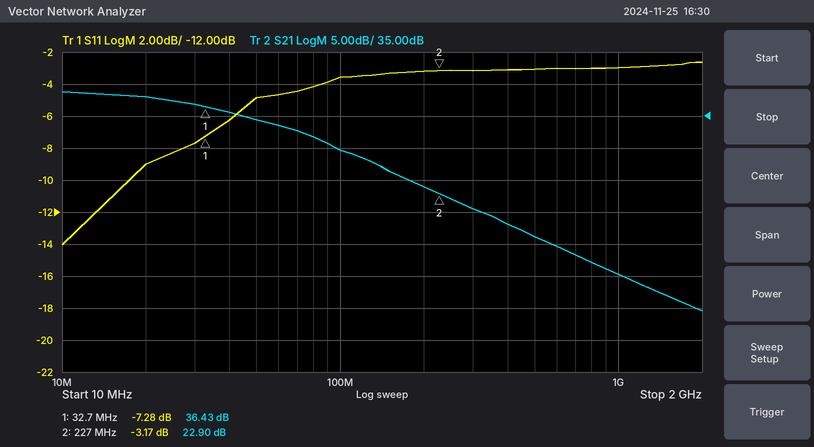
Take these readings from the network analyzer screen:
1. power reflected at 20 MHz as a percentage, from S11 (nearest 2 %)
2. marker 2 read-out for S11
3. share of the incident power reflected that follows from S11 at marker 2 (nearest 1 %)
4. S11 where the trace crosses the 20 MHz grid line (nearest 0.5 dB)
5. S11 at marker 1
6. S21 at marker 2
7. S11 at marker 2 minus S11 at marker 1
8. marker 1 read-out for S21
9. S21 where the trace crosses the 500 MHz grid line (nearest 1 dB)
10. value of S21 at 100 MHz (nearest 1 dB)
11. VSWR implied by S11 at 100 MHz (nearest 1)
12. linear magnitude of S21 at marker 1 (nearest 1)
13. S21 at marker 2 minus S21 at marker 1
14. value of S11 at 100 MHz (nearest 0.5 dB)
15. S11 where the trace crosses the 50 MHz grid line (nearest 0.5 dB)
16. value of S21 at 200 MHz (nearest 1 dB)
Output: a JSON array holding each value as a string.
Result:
["12 %", "-3.17 dB", "48 %", "-9.0 dB", "-7.28 dB", "22.90 dB", "4.11 dB", "36.43 dB", "16 dB", "30 dB", "5", "66", "-13.53 dB", "-3.5 dB", "-5.0 dB", "24 dB"]
